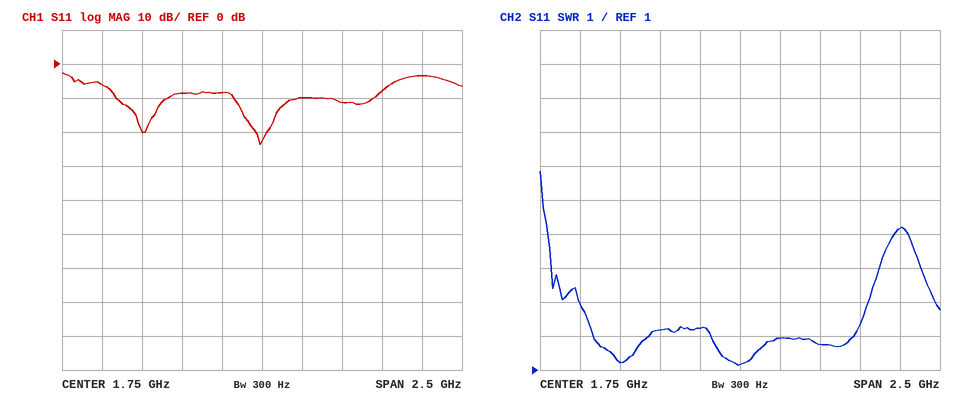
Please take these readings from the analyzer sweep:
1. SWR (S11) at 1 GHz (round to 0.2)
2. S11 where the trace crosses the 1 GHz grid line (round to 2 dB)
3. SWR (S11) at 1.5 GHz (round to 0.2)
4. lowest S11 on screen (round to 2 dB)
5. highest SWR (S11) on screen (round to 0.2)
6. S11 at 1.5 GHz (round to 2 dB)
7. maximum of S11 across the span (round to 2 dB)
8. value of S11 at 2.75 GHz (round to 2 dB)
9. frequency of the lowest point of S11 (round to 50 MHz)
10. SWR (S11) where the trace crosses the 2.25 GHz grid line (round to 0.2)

1.2
-20 dB
2.2
-24 dB
6.8
-8 dB
-2 dB
-4 dB
1.75 GHz
1.8
